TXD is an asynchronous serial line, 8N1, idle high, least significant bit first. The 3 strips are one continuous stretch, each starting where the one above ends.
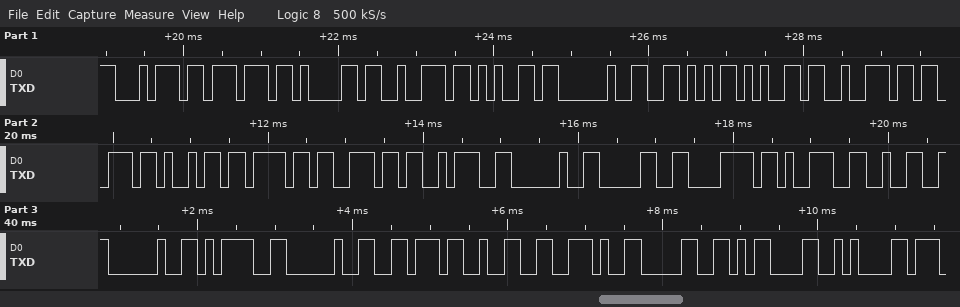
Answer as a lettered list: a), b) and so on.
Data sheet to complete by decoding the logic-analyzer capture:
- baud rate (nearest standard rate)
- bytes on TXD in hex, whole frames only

a) 9600 baud
b) 74 77 61 72 65 20 56 65 72 73 69 6F 6E 3A 20 30 78 39 32 20 3D 20 76 32 2E 30 0D 0A
